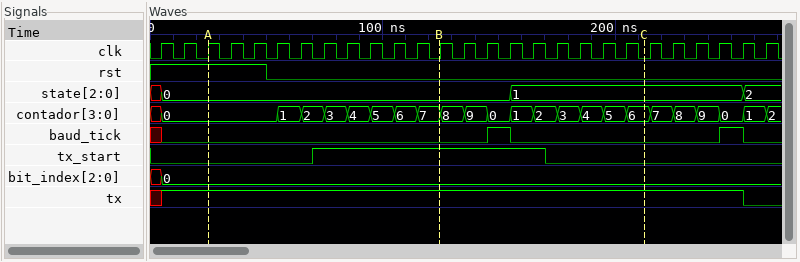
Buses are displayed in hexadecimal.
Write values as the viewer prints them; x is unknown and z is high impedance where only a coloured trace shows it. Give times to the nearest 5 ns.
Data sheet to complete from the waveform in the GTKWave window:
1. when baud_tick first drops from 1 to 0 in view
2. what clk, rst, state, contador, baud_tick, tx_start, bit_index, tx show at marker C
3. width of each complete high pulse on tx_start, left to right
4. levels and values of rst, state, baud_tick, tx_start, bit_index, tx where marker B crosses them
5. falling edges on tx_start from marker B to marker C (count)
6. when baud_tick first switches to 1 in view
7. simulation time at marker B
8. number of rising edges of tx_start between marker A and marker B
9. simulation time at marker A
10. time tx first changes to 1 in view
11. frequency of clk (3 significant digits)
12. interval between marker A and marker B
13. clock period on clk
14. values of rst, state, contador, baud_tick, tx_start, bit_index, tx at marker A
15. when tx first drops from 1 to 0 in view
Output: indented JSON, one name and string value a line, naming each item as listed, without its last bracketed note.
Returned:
{
  "when baud_tick first drops from 1 to 0 in view": "155 ns",
  "what clk, rst, state, contador, baud_tick, tx_start, bit_index, tx show at marker C": "clk=0, rst=0, state=1, contador=6, baud_tick=0, tx_start=0, bit_index=0, tx=1",
  "width of each complete high pulse on tx_start, left to right": "100 ns",
  "levels and values of rst, state, baud_tick, tx_start, bit_index, tx where marker B crosses them": "rst=0, state=0, baud_tick=0, tx_start=1, bit_index=0, tx=1",
  "falling edges on tx_start from marker B to marker C": "1",
  "when baud_tick first switches to 1 in view": "145 ns",
  "simulation time at marker B": "125 ns",
  "number of rising edges of tx_start between marker A and marker B": "1",
  "simulation time at marker A": "25 ns",
  "time tx first changes to 1 in view": "5 ns",
  "frequency of clk": "100 MHz",
  "interval between marker A and marker B": "100 ns",
  "clock period on clk": "10 ns",
  "values of rst, state, contador, baud_tick, tx_start, bit_index, tx at marker A": "rst=1, state=0, contador=0, baud_tick=0, tx_start=0, bit_index=0, tx=1",
  "when tx first drops from 1 to 0 in view": "255 ns"
}
